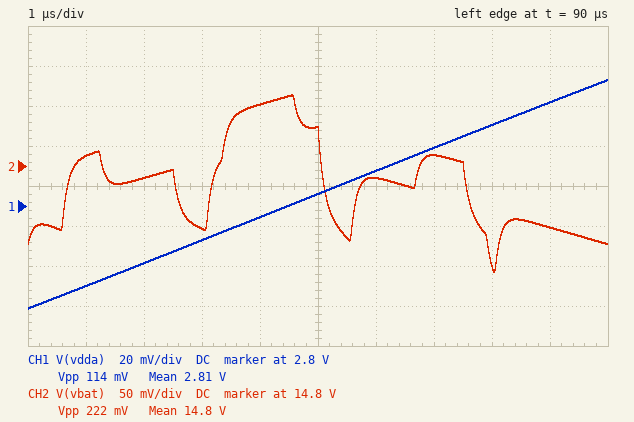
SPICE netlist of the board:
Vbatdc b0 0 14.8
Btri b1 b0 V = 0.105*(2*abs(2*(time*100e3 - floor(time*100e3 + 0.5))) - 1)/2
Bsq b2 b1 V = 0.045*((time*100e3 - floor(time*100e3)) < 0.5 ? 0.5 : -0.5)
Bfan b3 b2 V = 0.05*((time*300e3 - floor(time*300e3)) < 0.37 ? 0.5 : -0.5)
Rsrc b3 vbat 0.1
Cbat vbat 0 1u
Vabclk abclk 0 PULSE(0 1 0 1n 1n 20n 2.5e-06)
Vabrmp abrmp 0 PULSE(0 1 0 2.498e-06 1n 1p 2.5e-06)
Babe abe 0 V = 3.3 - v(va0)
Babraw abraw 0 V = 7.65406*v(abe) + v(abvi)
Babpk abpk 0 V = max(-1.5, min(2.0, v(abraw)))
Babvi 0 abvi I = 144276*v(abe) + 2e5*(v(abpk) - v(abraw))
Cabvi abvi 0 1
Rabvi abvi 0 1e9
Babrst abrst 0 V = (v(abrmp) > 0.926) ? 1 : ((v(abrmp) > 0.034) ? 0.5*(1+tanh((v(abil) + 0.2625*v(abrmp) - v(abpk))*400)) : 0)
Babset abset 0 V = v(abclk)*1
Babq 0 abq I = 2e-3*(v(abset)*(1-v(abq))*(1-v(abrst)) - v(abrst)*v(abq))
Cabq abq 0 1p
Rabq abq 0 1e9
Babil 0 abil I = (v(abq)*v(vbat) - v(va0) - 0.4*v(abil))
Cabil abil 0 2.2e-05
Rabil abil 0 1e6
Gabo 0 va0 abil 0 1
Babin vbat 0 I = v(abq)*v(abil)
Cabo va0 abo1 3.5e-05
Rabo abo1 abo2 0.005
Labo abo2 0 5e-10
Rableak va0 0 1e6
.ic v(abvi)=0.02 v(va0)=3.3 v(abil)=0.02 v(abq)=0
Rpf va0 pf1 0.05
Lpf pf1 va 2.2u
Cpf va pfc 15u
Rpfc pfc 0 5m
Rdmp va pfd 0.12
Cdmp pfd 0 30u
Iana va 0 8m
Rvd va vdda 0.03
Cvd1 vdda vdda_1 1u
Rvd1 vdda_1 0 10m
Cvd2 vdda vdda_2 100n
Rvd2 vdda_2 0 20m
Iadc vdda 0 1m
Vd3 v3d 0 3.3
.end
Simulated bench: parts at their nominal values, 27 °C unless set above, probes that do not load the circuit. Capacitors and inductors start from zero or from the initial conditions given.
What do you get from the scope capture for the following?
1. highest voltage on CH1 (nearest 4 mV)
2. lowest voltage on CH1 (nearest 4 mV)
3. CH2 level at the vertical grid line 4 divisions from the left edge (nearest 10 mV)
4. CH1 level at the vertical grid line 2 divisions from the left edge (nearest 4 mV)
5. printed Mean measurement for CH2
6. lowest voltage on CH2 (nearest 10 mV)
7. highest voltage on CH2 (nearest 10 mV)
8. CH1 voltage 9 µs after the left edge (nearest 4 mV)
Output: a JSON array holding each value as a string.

["2.864 V", "2.748 V", "14.88 V", "2.772 V", "14.8 V", "14.67 V", "14.89 V", "2.852 V"]
